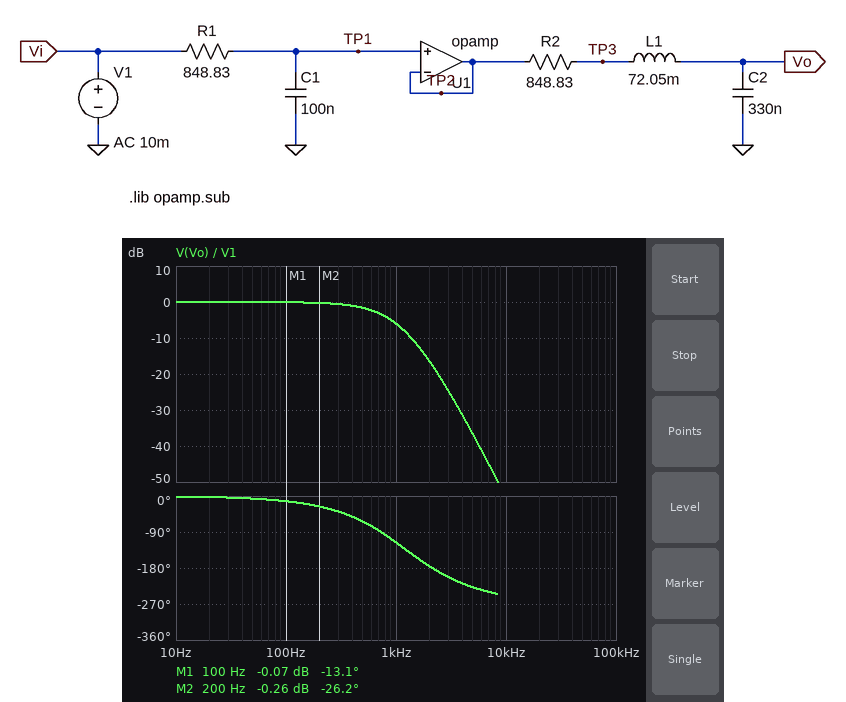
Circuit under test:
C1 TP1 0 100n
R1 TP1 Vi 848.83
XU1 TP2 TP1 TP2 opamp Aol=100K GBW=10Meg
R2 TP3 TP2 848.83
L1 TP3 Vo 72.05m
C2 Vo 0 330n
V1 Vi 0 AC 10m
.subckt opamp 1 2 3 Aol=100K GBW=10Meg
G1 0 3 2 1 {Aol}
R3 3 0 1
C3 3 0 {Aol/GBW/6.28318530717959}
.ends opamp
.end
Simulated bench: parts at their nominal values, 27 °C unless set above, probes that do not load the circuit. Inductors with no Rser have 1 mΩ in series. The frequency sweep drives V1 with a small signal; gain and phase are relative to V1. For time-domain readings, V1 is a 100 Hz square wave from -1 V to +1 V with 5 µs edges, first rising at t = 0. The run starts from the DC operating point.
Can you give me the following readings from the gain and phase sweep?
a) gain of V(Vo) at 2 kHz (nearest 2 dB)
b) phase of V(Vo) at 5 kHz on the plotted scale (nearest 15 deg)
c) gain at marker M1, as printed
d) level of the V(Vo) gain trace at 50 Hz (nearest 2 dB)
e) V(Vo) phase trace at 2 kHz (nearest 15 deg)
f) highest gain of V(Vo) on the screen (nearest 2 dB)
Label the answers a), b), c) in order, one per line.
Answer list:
a) -16 dB
b) -225 deg
c) -0.07 dB
d) 0 dB
e) -180 deg
f) 0 dB
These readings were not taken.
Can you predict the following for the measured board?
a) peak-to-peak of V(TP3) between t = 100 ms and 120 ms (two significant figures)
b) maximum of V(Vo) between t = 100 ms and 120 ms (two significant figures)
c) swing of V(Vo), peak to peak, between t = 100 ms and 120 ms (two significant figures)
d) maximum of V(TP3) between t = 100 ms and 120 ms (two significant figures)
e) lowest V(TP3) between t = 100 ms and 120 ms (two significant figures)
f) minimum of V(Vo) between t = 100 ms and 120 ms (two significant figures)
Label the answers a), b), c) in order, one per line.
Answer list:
a) 2.0 V
b) 1.0 V
c) 2.0 V
d) 1.0 V
e) -1.0 V
f) -1.0 V
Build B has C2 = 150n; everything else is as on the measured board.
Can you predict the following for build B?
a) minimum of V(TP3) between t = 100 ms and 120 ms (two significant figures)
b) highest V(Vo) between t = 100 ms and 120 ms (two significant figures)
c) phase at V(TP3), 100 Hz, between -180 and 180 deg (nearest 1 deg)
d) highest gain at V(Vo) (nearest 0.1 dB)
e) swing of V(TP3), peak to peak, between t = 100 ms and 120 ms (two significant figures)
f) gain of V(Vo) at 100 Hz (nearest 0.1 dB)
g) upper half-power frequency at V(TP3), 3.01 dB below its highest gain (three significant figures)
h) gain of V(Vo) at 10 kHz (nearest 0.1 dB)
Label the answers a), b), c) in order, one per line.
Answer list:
a) -1.1 V
b) 1.1 V
c) -8 deg
d) 0 dB
e) 2.1 V
f) 0 dB
g) 779 Hz
h) -47.2 dB
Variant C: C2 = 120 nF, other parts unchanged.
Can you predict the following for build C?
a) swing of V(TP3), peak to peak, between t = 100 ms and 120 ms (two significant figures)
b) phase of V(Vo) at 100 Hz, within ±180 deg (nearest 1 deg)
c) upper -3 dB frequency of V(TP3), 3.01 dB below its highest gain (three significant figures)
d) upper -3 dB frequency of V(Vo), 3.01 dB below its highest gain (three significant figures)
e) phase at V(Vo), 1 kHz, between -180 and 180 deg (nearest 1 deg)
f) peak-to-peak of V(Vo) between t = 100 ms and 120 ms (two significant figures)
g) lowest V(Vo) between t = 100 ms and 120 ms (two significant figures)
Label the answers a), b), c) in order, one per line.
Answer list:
a) 2.2 V
b) -7 deg
c) 897 Hz
d) 1.65 kHz
e) -72 deg
f) 2.3 V
g) -1.1 V
